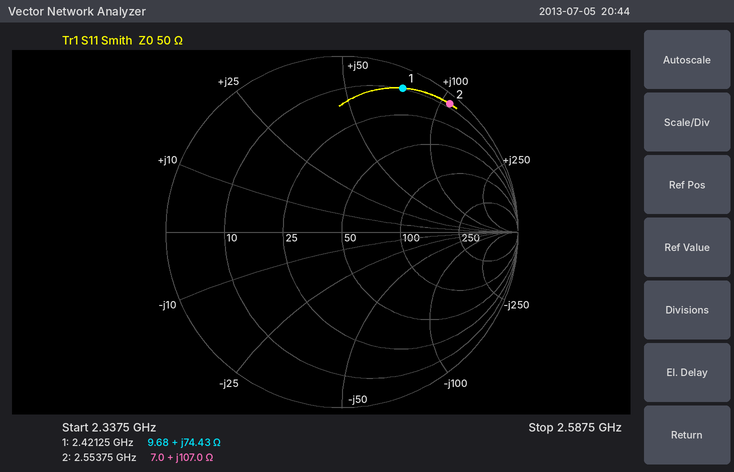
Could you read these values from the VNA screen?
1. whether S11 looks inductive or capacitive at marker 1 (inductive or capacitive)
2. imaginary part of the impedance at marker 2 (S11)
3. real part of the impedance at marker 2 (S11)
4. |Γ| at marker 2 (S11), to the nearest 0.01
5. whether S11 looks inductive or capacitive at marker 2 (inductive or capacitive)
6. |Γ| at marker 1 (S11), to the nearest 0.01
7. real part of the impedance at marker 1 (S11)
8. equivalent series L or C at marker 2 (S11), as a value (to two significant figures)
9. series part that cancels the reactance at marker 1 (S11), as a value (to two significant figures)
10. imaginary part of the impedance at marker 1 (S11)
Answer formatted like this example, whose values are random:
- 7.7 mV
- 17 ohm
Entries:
- inductive
- +107.0 Ω
- 7.0 Ω
- 0.95
- inductive
- 0.89
- 9.68 Ω
- 6.7 nH
- 880 fF
- +74.43 Ω
